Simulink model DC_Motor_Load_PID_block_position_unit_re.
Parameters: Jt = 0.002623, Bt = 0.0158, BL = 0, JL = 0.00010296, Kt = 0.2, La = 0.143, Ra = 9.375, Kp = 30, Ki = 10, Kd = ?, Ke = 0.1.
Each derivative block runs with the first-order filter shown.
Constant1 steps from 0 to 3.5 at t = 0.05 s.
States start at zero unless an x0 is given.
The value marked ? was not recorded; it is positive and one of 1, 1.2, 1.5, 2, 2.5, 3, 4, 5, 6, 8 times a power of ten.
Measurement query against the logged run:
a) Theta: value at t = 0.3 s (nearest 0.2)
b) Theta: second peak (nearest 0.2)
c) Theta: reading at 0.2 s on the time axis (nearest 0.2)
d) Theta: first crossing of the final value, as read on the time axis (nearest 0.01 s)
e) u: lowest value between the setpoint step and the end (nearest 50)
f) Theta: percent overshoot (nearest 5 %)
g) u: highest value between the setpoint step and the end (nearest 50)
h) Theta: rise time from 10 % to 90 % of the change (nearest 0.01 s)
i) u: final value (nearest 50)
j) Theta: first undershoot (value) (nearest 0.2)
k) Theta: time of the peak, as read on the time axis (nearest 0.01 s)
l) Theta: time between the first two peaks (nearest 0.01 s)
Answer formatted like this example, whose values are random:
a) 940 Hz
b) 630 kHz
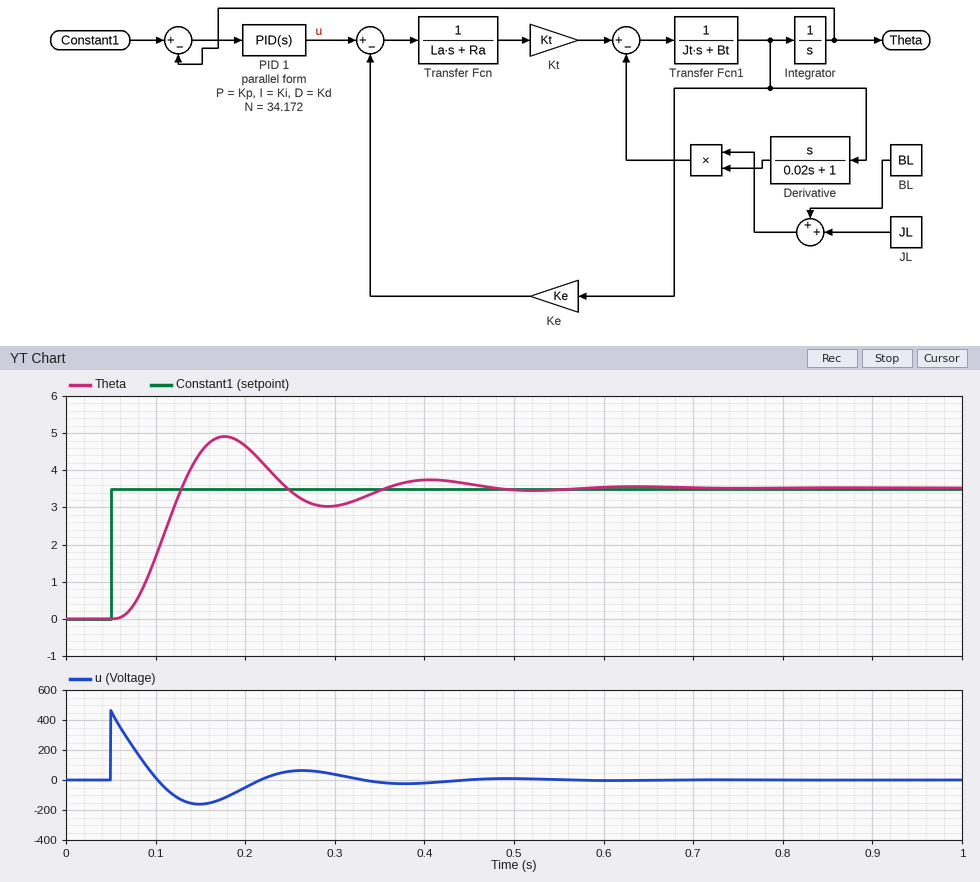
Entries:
a) 3.0
b) 3.8
c) 4.6
d) 0.13 s
e) -150
f) 40 %
g) 450
h) 0.05 s
i) 0
j) 3.0
k) 0.18 s
l) 0.23 s
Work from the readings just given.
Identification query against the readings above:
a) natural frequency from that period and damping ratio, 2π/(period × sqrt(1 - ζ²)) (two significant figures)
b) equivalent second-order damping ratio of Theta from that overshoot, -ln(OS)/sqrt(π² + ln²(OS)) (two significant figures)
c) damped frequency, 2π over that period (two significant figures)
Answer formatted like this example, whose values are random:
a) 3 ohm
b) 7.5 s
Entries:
a) 28 rad/s
b) 0.28
c) 27 rad/s
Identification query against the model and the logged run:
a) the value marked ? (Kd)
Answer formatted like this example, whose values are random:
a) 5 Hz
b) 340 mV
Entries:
a) 3
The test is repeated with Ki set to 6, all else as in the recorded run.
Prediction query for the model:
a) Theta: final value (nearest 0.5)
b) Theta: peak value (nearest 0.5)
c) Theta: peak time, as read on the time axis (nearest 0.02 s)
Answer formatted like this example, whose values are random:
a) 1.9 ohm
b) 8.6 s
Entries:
a) 3.5
b) 5.0
c) 0.18 s
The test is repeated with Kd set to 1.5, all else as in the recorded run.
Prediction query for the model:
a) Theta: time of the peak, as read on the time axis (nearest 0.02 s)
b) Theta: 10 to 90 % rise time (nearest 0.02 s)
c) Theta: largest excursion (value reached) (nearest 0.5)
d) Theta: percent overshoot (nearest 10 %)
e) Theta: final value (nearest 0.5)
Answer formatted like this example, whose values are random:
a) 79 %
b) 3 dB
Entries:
a) 0.22 s
b) 0.06 s
c) 5.0
d) 40 %
e) 3.5
